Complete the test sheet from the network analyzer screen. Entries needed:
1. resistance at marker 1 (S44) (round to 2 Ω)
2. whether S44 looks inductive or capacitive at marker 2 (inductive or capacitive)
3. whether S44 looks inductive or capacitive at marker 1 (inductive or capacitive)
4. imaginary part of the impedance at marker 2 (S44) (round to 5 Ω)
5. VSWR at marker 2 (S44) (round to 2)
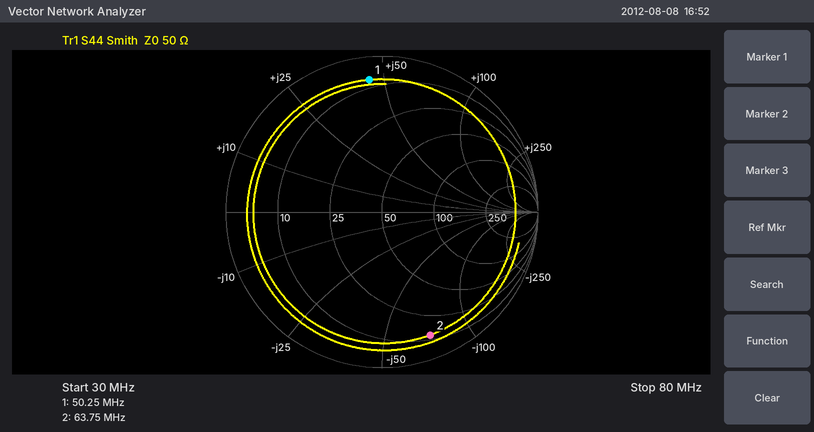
8 Ω
capacitive
inductive
-70 Ω
12
